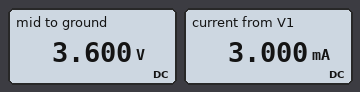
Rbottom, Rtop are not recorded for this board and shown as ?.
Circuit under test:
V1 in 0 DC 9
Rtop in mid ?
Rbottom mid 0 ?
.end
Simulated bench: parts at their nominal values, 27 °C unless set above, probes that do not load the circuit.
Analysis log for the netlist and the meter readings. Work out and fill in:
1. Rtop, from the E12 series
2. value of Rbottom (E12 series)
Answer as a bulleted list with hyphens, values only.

- 1.8 kΩ
- 1.2 kΩ
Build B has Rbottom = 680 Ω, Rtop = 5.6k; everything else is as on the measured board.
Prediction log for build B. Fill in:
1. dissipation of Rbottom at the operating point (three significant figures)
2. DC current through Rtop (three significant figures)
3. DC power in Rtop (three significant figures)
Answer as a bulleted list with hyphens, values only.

- 1.40 mW
- 1.43 mA
- 11.5 mW
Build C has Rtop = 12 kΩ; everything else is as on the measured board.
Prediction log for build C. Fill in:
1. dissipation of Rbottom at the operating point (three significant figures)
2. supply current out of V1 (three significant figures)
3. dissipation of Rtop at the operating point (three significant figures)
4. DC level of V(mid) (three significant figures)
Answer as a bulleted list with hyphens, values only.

- 558 µW
- 682 µA
- 5.58 mW
- 818 mV
